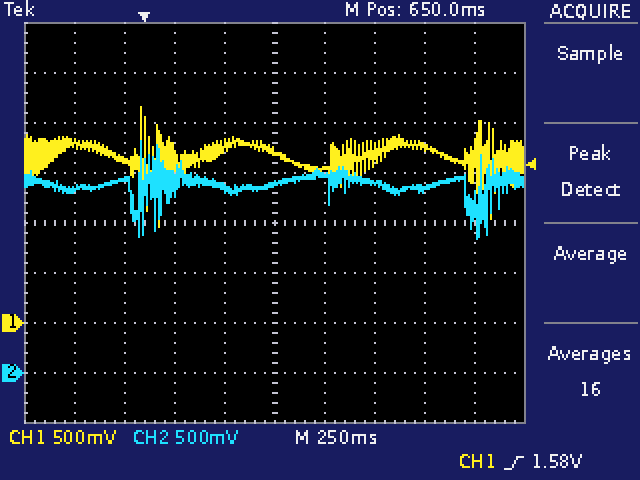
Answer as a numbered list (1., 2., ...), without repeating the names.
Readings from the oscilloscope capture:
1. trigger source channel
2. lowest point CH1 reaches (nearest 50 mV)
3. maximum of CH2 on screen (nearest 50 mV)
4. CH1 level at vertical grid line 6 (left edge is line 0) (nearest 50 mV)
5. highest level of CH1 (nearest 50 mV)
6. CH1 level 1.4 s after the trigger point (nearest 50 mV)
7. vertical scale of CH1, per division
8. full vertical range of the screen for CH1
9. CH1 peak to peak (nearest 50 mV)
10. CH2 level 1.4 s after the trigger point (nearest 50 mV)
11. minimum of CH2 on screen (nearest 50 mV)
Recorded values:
1. CH1
2. 950 mV
3. 2.30 V
4. 1.55 V
5. 2.15 V
6. 1.75 V
7. 500 mV
8. 4 V
9. 1.20 V
10. 1.85 V
11. 1.35 V
